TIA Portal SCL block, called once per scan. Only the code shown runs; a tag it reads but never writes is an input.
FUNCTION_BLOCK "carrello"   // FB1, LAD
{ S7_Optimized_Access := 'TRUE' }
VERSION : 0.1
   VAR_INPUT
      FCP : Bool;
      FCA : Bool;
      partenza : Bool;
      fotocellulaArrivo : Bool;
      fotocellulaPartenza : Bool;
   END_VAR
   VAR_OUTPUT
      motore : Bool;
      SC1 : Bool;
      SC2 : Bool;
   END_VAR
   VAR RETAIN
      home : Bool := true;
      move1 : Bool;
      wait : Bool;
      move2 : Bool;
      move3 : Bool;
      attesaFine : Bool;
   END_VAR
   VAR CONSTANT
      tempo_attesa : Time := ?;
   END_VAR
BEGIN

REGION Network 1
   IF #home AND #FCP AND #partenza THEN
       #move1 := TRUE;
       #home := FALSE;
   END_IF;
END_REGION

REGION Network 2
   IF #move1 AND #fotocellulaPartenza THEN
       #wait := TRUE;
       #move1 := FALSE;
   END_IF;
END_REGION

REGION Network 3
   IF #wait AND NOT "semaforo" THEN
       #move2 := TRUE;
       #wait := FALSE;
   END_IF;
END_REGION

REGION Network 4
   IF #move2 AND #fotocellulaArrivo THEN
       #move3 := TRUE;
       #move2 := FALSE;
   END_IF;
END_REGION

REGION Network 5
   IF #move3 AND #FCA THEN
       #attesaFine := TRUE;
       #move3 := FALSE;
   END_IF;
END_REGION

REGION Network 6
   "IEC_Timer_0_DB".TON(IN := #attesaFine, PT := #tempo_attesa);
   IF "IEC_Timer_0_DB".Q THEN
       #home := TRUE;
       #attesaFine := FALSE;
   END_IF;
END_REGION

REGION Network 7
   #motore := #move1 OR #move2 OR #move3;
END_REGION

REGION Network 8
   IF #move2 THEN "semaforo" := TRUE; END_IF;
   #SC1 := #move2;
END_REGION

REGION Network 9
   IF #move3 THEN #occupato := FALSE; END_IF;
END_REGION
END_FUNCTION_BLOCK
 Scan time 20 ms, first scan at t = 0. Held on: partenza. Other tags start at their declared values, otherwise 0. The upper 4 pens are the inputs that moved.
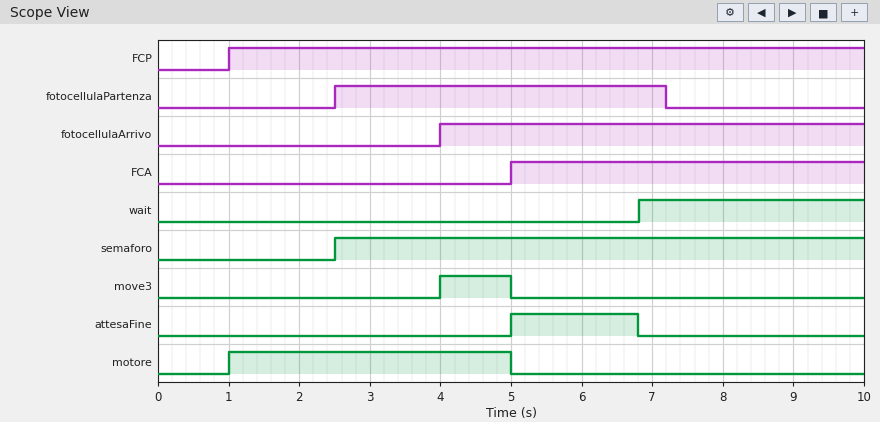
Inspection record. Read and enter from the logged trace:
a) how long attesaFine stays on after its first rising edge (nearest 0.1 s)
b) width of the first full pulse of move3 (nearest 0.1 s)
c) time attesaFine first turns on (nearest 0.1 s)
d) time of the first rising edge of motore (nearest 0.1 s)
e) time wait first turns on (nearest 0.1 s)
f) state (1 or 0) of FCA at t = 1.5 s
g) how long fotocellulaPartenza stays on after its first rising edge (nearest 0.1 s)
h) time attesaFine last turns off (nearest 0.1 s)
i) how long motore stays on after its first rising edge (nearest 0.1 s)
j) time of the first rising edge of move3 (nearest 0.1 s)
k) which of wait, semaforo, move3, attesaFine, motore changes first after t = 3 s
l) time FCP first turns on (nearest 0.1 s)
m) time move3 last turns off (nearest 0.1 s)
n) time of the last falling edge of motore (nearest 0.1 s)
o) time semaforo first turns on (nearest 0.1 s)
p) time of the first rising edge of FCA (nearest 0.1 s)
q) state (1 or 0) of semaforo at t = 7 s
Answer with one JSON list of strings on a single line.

["1.8 s", "1.0 s", "5.0 s", "1.0 s", "6.8 s", "0", "4.7 s", "6.8 s", "4.0 s", "4.0 s", "move3", "1.0 s", "5.0 s", "5.0 s", "2.5 s", "5.0 s", "1"]
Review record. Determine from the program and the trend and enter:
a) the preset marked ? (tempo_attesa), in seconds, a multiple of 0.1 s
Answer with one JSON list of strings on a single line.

["1.8 s"]
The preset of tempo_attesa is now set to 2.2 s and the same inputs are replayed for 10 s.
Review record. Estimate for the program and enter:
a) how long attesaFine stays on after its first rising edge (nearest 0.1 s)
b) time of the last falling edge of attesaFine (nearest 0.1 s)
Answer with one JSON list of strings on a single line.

["2.2 s", "7.2 s"]
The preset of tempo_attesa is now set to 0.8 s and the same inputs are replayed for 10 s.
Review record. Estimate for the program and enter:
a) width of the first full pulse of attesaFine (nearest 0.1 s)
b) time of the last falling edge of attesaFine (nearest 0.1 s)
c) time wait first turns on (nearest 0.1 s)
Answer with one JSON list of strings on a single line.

["0.8 s", "5.8 s", "5.8 s"]
